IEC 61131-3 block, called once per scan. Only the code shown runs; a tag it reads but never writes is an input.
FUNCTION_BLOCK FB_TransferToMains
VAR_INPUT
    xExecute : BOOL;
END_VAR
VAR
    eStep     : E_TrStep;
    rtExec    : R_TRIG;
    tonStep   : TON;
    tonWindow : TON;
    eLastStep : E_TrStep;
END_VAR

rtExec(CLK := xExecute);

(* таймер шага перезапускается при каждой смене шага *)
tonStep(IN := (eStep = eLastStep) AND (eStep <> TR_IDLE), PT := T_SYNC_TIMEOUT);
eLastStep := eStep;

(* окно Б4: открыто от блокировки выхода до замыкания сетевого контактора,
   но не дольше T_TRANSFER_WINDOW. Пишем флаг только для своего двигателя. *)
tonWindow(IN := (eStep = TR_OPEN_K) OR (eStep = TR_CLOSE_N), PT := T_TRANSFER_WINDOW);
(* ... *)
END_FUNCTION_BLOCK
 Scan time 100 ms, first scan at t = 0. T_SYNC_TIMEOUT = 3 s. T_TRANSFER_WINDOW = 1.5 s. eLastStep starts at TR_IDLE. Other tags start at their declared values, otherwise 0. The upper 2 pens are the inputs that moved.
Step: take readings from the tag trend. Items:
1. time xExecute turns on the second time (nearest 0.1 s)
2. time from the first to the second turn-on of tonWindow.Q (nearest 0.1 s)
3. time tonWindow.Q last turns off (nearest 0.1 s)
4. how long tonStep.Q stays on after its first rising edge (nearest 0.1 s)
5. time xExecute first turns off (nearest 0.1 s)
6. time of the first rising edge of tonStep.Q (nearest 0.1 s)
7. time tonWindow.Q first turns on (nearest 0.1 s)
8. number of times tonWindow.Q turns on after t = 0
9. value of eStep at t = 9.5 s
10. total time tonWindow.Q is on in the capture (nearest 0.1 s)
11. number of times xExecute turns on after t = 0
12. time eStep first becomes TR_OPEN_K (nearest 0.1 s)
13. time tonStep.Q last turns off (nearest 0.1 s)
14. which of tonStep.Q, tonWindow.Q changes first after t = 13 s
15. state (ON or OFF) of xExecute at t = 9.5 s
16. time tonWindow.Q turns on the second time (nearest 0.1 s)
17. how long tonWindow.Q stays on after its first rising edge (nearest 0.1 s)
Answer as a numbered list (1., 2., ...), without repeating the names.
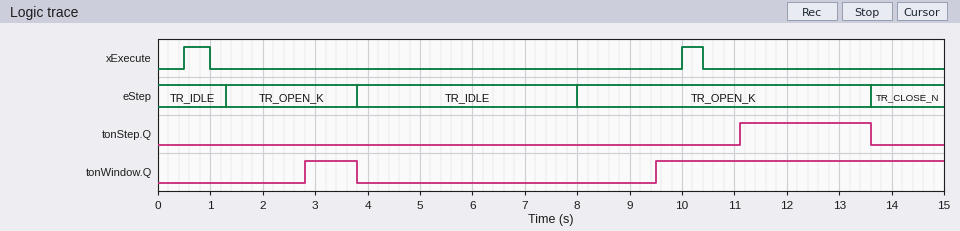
1. 10.0 s
2. 6.7 s
3. 3.8 s
4. 2.5 s
5. 1.0 s
6. 11.1 s
7. 2.8 s
8. 2
9. TR_OPEN_K
10. 6.5 s
11. 2
12. 1.3 s
13. 13.6 s
14. tonStep.Q
15. OFF
16. 9.5 s
17. 1.0 s
